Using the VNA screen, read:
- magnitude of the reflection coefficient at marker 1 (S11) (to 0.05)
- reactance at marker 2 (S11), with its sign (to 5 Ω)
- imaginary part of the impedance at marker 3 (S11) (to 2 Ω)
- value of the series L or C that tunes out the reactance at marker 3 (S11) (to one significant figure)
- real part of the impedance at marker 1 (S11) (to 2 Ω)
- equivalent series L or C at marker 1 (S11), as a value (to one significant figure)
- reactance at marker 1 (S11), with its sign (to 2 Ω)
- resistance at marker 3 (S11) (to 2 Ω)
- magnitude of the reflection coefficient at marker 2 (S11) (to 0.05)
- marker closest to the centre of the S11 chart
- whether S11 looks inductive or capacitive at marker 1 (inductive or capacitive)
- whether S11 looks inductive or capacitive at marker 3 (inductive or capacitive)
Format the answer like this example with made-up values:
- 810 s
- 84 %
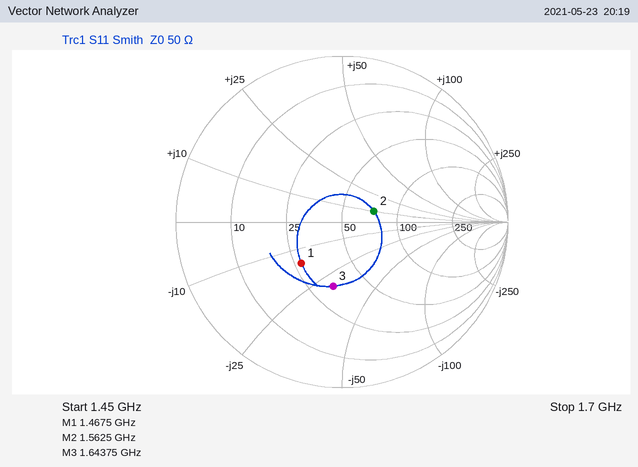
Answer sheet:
- 0.35
- +10 Ω
- -30 Ω
- 3 nH
- 28 Ω
- 7 pF
- -16 Ω
- 34 Ω
- 0.20
- marker 2
- capacitive
- capacitive
